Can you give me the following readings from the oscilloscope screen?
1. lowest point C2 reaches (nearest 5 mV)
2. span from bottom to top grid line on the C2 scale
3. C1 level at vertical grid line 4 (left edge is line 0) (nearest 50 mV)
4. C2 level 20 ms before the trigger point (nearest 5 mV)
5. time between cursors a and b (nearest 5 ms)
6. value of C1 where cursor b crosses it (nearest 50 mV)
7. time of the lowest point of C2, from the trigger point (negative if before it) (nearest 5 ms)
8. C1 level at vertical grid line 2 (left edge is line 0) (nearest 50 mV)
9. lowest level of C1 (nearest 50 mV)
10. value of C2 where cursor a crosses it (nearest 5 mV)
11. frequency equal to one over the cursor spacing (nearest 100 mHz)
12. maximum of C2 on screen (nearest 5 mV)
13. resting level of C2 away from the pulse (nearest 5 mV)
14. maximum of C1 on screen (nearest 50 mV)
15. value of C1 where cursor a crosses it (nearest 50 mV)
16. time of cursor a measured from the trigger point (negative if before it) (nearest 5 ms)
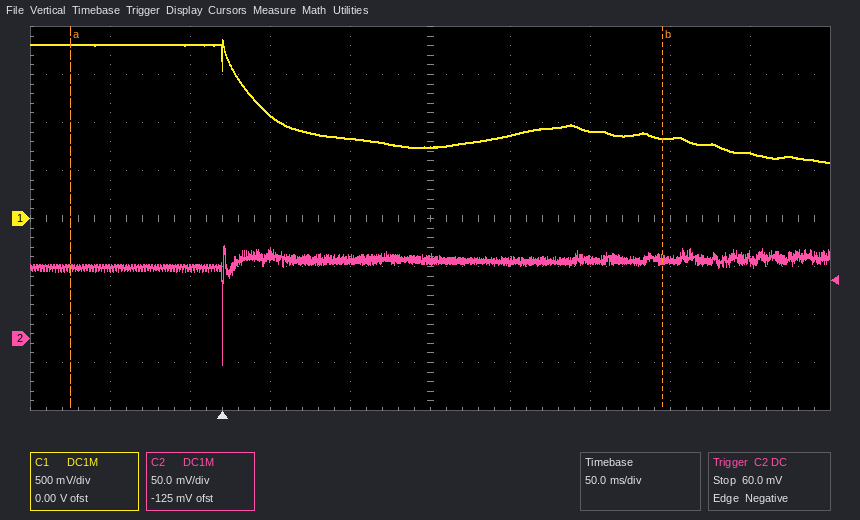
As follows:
-25 mV
400 mV
850 mV
75 mV
370 ms
850 mV
0 ms
1.80 V
600 mV
75 mV
2.7 Hz
95 mV
80 mV
1.85 V
1.80 V
-95 ms
